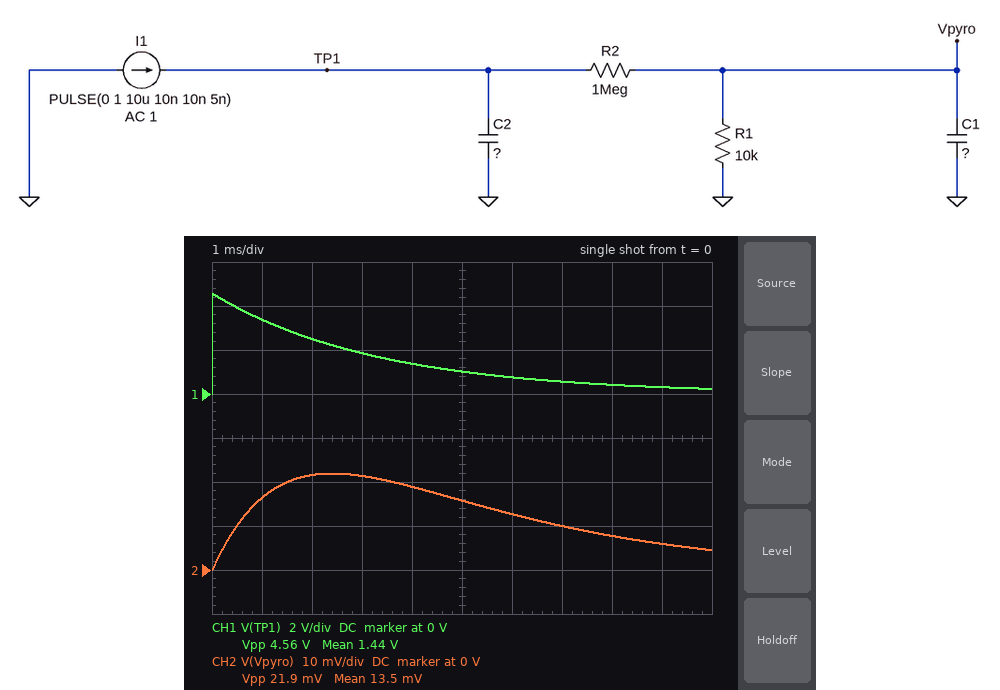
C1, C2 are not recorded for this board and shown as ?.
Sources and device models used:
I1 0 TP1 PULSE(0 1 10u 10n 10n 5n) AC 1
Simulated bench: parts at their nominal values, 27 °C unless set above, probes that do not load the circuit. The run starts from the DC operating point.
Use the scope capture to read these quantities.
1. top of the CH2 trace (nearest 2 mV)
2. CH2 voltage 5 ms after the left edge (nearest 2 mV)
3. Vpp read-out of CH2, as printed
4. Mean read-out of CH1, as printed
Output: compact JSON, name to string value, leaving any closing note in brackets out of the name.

{"top of the CH2 trace": "22 mV", "CH2 voltage 5 ms after the left edge": "16 mV", "Vpp read-out of CH2, as printed": "21.9 mV", "Mean read-out of CH1, as printed": "1.44 V"}
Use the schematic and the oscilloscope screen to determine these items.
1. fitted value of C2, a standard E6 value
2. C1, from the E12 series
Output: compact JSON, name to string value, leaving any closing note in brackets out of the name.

{"fitted value of C2, a standard E6 value": "3.3 nF", "C1, from the E12 series": "180 nF"}
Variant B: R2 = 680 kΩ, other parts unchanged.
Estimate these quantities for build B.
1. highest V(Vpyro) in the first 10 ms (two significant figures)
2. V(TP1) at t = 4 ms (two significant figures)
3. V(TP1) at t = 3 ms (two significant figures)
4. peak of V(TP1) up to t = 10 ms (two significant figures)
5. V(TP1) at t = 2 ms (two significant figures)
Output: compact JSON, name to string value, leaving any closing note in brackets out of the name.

{"highest V(Vpyro) in the first 10 ms": "27 mV", "V(TP1) at t = 4 ms": "790 mV", "V(TP1) at t = 3 ms": "1.2 V", "peak of V(TP1) up to t = 10 ms": "4.6 V", "V(TP1) at t = 2 ms": "1.9 V"}
